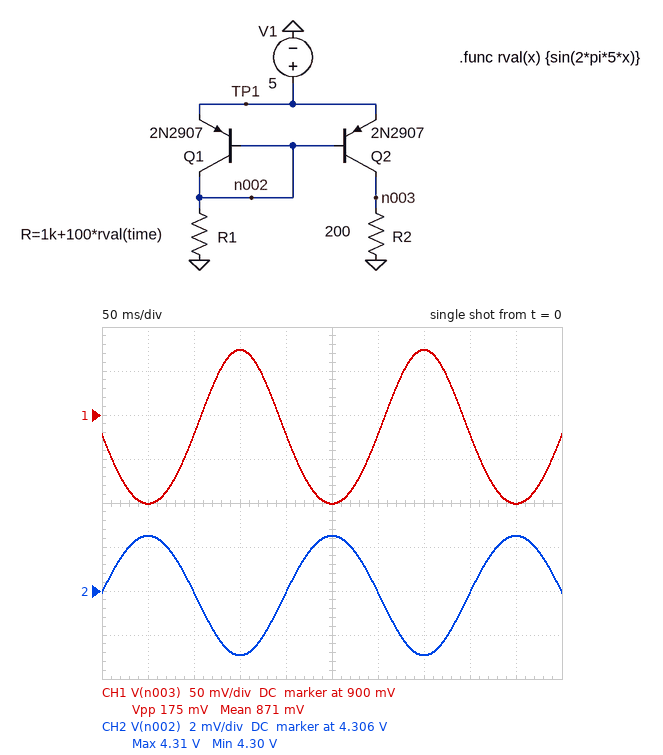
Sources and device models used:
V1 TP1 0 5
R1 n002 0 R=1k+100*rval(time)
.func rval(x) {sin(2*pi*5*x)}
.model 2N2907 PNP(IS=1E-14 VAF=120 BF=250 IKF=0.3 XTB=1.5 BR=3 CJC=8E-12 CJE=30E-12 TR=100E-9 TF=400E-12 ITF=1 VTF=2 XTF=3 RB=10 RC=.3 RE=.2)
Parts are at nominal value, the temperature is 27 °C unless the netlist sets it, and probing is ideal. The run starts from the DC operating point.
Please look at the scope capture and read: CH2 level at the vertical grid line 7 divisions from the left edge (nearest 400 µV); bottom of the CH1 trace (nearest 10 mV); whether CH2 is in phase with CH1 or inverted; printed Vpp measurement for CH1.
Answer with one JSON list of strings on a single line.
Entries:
["4.3032 V", "800 mV", "inverted", "175 mV"]
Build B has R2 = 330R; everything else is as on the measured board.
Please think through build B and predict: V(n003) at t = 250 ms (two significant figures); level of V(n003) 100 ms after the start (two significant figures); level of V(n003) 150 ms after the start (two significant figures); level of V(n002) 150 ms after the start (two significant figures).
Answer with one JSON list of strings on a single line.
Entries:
["1.3 V", "1.4 V", "1.6 V", "4.3 V"]
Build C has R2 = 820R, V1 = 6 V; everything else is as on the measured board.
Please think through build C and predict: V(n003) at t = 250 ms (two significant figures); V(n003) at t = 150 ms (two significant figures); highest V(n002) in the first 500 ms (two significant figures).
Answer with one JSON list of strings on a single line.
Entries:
["4.0 V", "4.8 V", "5.3 V"]
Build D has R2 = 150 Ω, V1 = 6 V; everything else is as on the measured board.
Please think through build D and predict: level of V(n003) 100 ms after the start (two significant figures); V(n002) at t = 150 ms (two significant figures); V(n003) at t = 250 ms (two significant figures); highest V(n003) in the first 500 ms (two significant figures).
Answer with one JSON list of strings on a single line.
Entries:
["820 mV", "5.3 V", "740 mV", "910 mV"]
